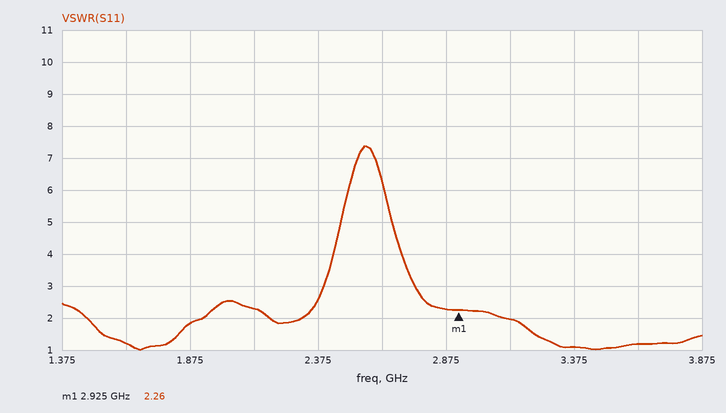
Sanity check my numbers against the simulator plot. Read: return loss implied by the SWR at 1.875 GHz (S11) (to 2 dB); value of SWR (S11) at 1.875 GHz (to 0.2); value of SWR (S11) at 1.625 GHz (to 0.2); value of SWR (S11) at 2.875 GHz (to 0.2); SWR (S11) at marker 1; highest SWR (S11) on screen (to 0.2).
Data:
10 dB
1.8
1.2
2.2
2.26
7.4
